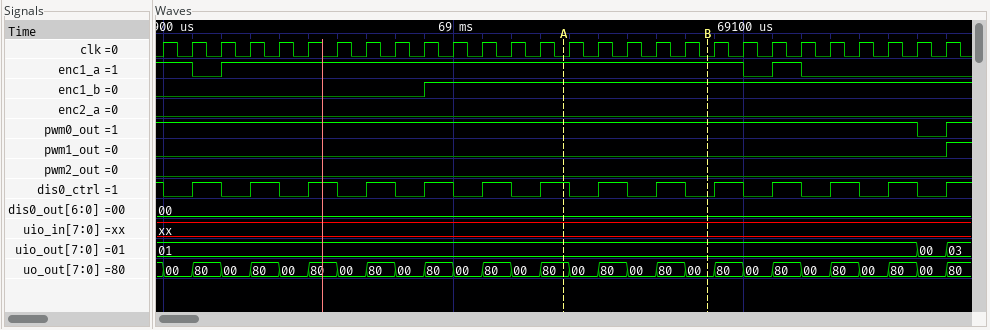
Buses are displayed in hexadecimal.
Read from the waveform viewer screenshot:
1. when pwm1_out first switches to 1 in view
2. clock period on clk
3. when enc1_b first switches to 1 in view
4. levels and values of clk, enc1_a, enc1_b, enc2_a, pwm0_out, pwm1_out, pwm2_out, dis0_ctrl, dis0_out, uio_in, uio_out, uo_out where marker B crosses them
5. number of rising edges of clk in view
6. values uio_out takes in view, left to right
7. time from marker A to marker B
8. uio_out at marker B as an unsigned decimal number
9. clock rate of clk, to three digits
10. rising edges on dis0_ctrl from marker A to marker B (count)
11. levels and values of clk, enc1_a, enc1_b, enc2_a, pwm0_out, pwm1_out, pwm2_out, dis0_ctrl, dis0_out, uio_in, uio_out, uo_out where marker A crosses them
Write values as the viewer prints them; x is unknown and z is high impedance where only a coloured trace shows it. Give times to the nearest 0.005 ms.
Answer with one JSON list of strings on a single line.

["69.17 ms", "0.01 ms", "68.99 ms", "clk=0, enc1_a=1, enc1_b=1, enc2_a=0, pwm0_out=1, pwm1_out=0, pwm2_out=0, dis0_ctrl=0, dis0_out=00, uio_in=xx, uio_out=01, uo_out=00", "28", "01, 00, 03", "0.05 ms", "1", "100 kHz", "2", "clk=0, enc1_a=1, enc1_b=1, enc2_a=0, pwm0_out=1, pwm1_out=0, pwm2_out=0, dis0_ctrl=1, dis0_out=00, uio_in=xx, uio_out=01, uo_out=80"]
